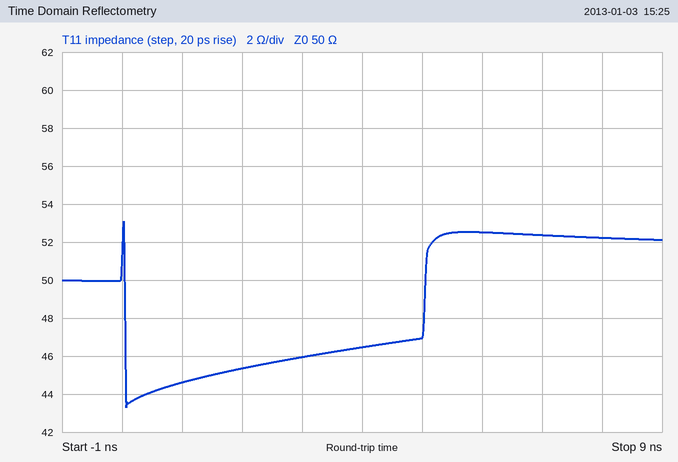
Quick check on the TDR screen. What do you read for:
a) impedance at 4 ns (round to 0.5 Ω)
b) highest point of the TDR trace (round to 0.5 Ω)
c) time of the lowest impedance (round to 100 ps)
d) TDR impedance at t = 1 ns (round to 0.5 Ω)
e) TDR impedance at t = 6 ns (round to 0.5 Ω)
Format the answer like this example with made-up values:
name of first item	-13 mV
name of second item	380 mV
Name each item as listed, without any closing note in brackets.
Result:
impedance at 4 ns	46.5 Ω
highest point of the TDR trace	53.0 Ω
time of the lowest impedance	100 ps
TDR impedance at t = 1 ns	44.5 Ω
TDR impedance at t = 6 ns	52.5 Ω
